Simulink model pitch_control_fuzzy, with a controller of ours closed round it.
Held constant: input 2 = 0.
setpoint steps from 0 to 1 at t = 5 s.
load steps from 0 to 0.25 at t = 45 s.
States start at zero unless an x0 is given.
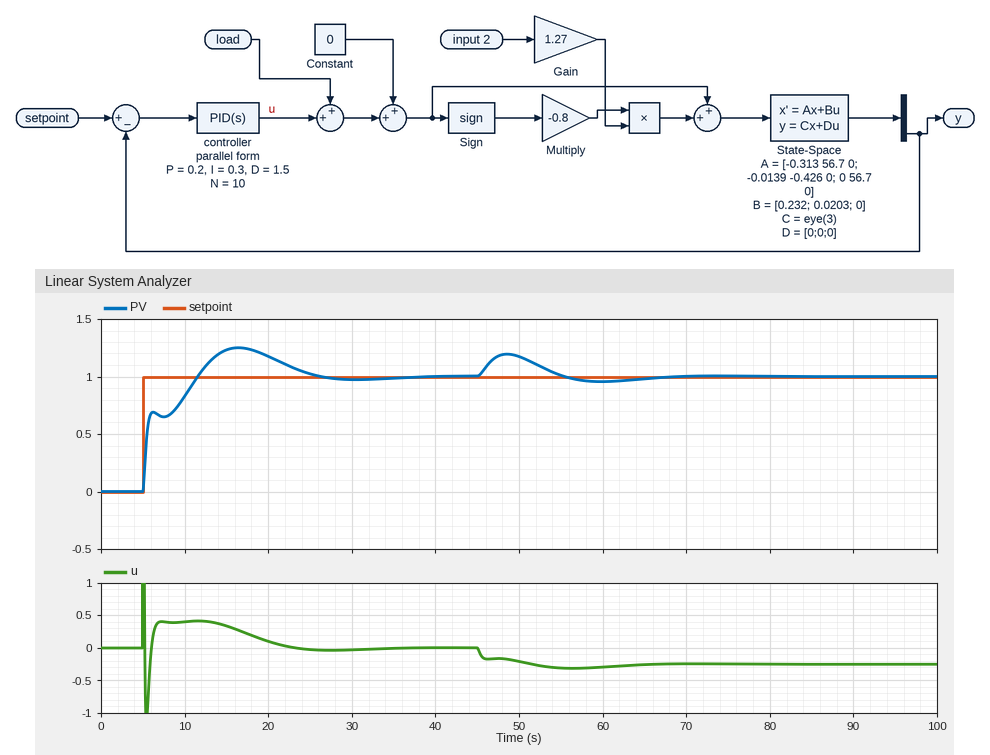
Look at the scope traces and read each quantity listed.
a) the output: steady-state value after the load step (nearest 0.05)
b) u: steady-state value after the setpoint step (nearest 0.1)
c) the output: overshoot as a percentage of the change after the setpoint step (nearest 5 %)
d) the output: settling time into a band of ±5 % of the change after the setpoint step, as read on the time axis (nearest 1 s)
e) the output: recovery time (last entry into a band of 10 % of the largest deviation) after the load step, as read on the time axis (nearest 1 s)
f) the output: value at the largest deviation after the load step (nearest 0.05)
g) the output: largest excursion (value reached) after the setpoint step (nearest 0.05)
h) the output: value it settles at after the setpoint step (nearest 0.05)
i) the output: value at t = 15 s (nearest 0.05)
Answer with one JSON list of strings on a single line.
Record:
["1.00", "0.0", "25 %", "24 s", "65 s", "1.20", "1.25", "1.00", "1.25"]
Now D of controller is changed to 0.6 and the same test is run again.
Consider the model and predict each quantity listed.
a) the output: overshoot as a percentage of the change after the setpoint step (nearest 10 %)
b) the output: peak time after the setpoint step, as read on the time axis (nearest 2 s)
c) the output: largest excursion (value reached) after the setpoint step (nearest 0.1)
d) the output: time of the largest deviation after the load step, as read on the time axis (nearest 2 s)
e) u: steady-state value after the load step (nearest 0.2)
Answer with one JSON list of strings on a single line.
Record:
["20 %", "14 s", "1.2", "48 s", "-0.2"]
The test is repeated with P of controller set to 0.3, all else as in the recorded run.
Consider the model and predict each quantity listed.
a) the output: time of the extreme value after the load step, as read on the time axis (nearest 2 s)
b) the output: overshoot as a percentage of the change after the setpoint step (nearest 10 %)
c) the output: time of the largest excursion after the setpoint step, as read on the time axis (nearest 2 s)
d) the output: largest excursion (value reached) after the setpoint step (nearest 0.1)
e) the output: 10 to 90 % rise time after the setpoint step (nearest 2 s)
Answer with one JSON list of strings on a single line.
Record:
["48 s", "20 %", "16 s", "1.2", "6 s"]
